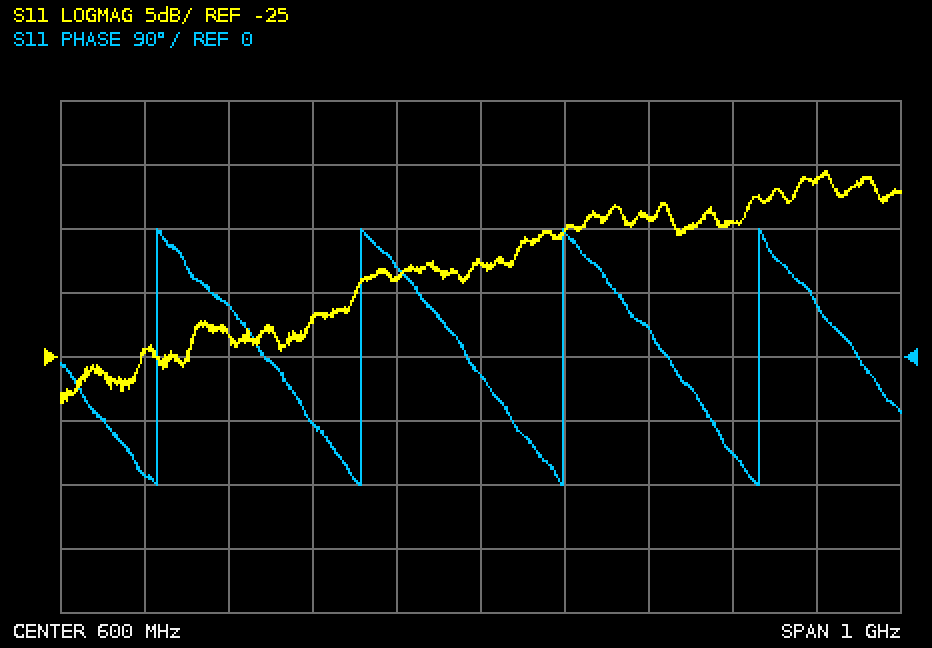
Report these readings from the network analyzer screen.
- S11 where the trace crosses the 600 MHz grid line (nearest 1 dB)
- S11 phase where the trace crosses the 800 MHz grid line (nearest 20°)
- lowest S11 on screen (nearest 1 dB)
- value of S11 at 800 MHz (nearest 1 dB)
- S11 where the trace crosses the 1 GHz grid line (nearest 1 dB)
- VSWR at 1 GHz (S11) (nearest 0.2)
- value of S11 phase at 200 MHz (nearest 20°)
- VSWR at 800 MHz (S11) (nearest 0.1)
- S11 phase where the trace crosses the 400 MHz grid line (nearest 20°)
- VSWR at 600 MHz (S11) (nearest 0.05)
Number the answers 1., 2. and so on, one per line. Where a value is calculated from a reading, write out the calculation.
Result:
1. -18 dB
2. 40°
3. -29 dB
4. -14 dB
5. -11 dB
6. |Γ| = 10^(-11/20) = 0.2818; VSWR = (1 + 0.2818)/(1 − 0.2818) ≈ 1.8
7. -160°
8. |Γ| = 10^(-14/20) = 0.1995; VSWR = (1 + 0.1995)/(1 − 0.1995) ≈ 1.5
9. -100°
10. |Γ| = 10^(-18/20) = 0.1259; VSWR = (1 + 0.1259)/(1 − 0.1259) ≈ 1.29, so 1.30 to the nearest 0.05
